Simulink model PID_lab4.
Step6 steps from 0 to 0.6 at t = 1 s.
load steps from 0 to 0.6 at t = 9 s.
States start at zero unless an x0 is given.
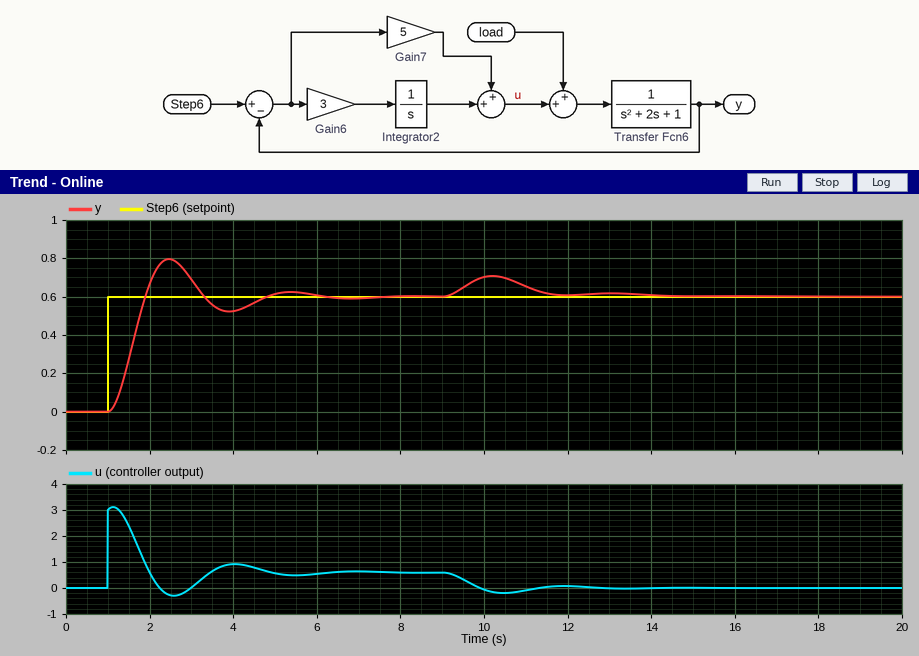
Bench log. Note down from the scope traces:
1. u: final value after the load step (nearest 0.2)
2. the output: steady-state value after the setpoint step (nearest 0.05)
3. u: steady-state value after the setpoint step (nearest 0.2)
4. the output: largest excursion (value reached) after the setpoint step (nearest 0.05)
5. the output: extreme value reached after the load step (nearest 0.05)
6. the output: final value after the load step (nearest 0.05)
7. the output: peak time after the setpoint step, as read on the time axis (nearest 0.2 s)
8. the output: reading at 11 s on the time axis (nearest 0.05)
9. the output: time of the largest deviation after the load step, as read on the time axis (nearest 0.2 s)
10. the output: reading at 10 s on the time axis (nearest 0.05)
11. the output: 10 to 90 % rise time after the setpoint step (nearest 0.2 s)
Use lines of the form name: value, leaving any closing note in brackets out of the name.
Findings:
u: final value after the load step: 0.0
the output: steady-state value after the setpoint step: 0.60
u: steady-state value after the setpoint step: 0.6
the output: largest excursion (value reached) after the setpoint step: 0.80
the output: extreme value reached after the load step: 0.70
the output: final value after the load step: 0.60
the output: peak time after the setpoint step, as read on the time axis: 2.4 s
the output: reading at 11 s on the time axis: 0.65
the output: time of the largest deviation after the load step, as read on the time axis: 10.2 s
the output: reading at 10 s on the time axis: 0.70
the output: 10 to 90 % rise time after the setpoint step: 0.6 s
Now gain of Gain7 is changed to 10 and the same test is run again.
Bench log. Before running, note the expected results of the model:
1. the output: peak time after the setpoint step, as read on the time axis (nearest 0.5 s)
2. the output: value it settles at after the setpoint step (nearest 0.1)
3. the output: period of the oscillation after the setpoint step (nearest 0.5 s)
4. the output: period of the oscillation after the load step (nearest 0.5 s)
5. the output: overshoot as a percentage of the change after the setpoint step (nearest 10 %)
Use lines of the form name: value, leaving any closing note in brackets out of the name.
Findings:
the output: peak time after the setpoint step, as read on the time axis: 2.0 s
the output: value it settles at after the setpoint step: 0.6
the output: period of the oscillation after the setpoint step: 2.0 s
the output: period of the oscillation after the load step: 2.0 s
the output: overshoot as a percentage of the change after the setpoint step: 40 %
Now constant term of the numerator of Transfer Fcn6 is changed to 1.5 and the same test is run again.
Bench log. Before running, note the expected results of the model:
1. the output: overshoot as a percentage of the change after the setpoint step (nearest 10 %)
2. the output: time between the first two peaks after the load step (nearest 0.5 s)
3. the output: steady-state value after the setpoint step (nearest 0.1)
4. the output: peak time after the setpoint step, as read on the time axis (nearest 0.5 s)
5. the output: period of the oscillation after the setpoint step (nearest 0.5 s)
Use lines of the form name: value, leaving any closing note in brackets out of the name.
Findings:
the output: overshoot as a percentage of the change after the setpoint step: 40 %
the output: time between the first two peaks after the load step: 2.5 s
the output: steady-state value after the setpoint step: 0.6
the output: peak time after the setpoint step, as read on the time axis: 2.0 s
the output: period of the oscillation after the setpoint step: 2.5 s
